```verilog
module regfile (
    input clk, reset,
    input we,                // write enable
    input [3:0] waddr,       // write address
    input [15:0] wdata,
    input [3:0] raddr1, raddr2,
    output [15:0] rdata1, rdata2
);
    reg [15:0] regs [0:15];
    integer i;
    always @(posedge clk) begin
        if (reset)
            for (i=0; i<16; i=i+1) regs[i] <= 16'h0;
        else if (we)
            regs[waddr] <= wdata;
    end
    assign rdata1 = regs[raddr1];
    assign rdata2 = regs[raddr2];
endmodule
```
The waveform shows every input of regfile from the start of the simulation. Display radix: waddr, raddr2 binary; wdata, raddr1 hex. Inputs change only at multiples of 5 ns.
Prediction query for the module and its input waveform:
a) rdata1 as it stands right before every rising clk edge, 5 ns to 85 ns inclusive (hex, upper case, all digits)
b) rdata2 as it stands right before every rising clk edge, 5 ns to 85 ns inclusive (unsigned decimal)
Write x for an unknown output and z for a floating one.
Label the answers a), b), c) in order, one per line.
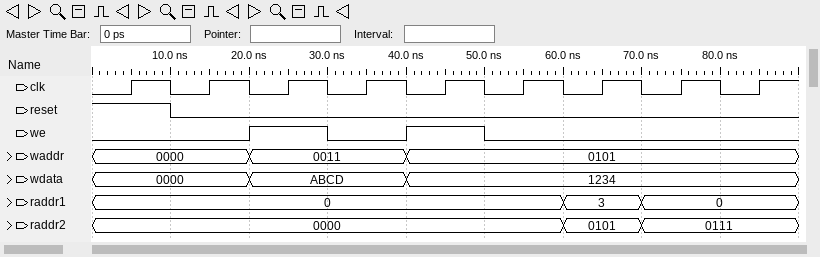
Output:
a) x, 0000, 0000, 0000, 0000, 0000, ABCD, 0000, 0000
b) x, 0, 0, 0, 0, 0, 4660, 0, 0
